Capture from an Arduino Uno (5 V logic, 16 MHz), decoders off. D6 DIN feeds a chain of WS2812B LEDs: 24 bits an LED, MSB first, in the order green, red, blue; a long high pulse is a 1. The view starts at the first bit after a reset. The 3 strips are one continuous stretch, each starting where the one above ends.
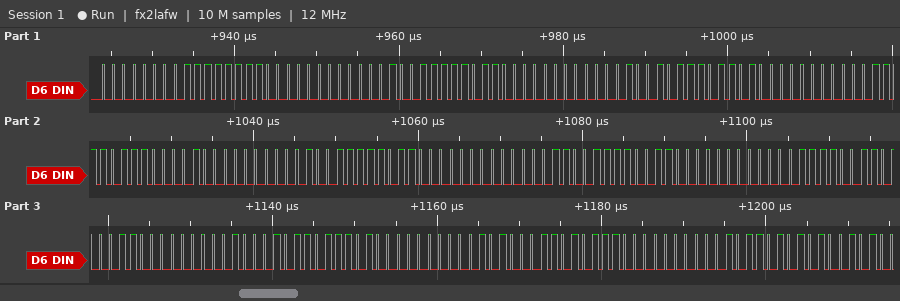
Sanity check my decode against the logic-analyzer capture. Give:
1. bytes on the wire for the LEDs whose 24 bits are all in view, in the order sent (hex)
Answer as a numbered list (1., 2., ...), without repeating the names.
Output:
1. 00 FF 00 09 F6 00 12 ED 00 1E E1 00 27 D8 00 33 CC 00 3C C3 00 45 BA 00 51 AE 00
